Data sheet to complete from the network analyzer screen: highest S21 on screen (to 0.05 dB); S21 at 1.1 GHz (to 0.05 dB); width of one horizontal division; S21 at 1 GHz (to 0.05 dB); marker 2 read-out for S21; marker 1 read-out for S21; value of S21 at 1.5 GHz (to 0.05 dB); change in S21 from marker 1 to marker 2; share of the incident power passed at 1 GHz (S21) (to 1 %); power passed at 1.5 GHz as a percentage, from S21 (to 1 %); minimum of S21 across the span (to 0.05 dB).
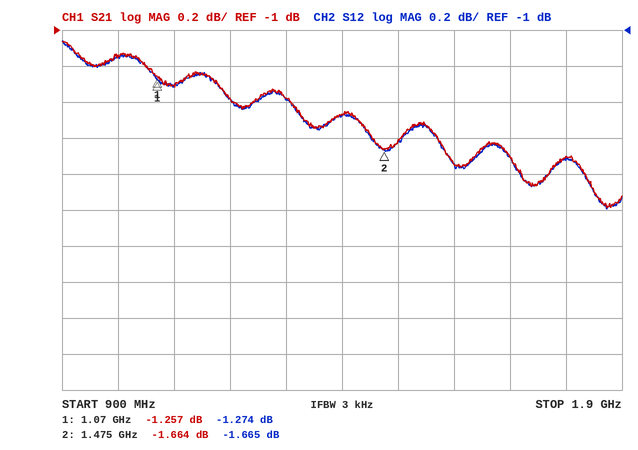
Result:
-1.05 dB
-1.30 dB
100 MHz
-1.15 dB
-1.664 dB
-1.257 dB
-1.60 dB
-0.407 dB
77 %
69 %
-2.00 dB
